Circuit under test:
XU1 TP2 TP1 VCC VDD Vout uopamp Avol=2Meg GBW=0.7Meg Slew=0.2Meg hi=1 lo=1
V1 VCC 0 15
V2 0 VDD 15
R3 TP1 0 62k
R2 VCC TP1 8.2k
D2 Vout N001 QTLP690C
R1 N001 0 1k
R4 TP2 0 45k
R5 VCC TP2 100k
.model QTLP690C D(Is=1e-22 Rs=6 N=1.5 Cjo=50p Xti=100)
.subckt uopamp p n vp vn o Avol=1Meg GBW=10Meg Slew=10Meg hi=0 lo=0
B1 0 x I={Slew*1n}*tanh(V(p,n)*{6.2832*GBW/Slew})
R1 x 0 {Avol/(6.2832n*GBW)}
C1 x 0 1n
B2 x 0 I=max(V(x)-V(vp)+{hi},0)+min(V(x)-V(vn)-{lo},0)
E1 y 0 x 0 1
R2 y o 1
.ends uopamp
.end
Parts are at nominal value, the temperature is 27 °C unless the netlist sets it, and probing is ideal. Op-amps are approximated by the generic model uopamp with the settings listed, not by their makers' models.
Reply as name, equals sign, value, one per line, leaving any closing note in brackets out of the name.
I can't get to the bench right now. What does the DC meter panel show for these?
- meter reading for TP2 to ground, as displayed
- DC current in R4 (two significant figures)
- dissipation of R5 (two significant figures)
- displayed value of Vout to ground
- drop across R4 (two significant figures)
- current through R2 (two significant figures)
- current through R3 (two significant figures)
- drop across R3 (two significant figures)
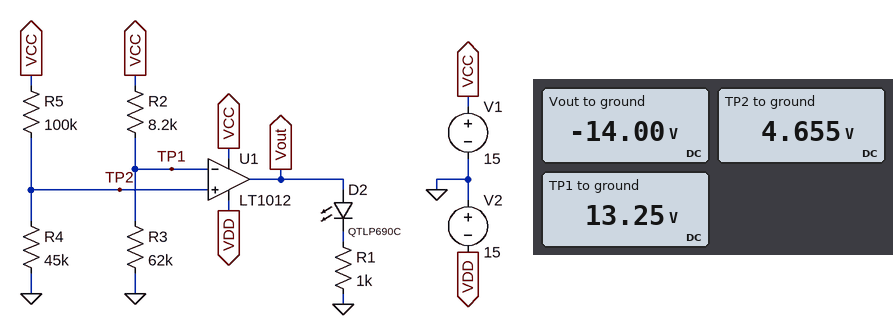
meter reading for TP2 to ground, as displayed = 4.655 V
DC current in R4 = 100 µA
dissipation of R5 = 1.1 mW
displayed value of Vout to ground = -14.00 V
drop across R4 = 4.7 V
current through R2 = 210 µA
current through R3 = 210 µA
drop across R3 = 13 V
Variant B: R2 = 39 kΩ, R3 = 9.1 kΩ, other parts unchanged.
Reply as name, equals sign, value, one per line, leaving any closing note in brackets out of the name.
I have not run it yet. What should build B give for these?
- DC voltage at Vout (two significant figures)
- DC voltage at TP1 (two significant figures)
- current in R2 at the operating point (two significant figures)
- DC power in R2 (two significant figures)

DC voltage at Vout = 14 V
DC voltage at TP1 = 2.8 V
current in R2 at the operating point = 310 µA
DC power in R2 = 3.8 mW
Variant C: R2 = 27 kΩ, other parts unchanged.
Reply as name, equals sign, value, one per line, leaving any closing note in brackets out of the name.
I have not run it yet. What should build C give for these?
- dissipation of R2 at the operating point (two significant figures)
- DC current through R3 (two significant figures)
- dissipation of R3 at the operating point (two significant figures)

dissipation of R2 at the operating point = 770 µW
DC current through R3 = 170 µA
dissipation of R3 at the operating point = 1.8 mW
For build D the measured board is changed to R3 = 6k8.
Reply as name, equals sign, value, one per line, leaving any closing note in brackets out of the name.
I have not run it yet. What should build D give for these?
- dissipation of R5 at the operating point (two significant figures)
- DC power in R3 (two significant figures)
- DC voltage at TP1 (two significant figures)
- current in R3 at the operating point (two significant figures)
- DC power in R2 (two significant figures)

dissipation of R5 at the operating point = 1.1 mW
DC power in R3 = 6.8 mW
DC voltage at TP1 = 6.8 V
current in R3 at the operating point = 1.0 mA
DC power in R2 = 8.2 mW
